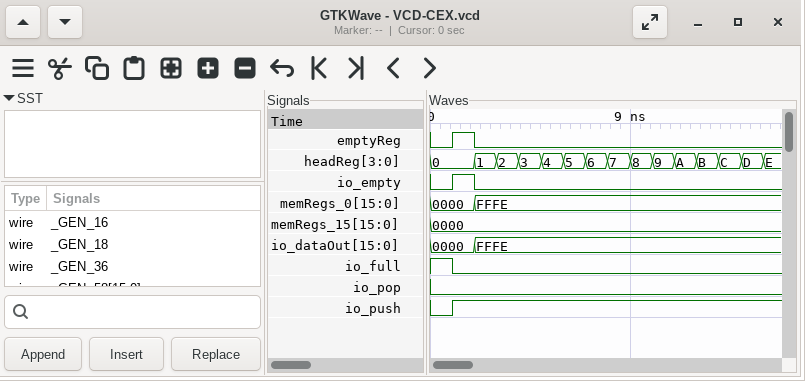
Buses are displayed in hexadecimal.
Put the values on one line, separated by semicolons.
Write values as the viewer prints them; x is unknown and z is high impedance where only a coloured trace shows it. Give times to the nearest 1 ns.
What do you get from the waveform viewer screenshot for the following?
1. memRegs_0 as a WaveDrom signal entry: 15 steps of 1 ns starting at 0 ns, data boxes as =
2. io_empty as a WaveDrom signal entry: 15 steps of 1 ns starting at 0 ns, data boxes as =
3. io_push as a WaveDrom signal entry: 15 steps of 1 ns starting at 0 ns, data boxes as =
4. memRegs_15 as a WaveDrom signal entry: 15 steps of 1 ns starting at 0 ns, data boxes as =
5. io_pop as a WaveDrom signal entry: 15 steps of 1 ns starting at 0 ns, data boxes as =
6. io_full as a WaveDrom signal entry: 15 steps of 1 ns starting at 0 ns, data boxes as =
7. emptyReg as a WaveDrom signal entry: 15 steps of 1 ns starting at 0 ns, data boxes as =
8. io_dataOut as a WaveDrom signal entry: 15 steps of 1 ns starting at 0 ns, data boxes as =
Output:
{name: 'memRegs_0', wave: '=.=............', data: '0000 FFFE'}; {name: 'io_empty', wave: '010............'}; {name: 'io_push', wave: '01.............'}; {name: 'memRegs_15', wave: '=..............', data: '0000'}; {name: 'io_pop', wave: '0..............'}; {name: 'io_full', wave: '10.............'}; {name: 'emptyReg', wave: '010............'}; {name: 'io_dataOut', wave: '=.=............', data: '0000 FFFE'}
